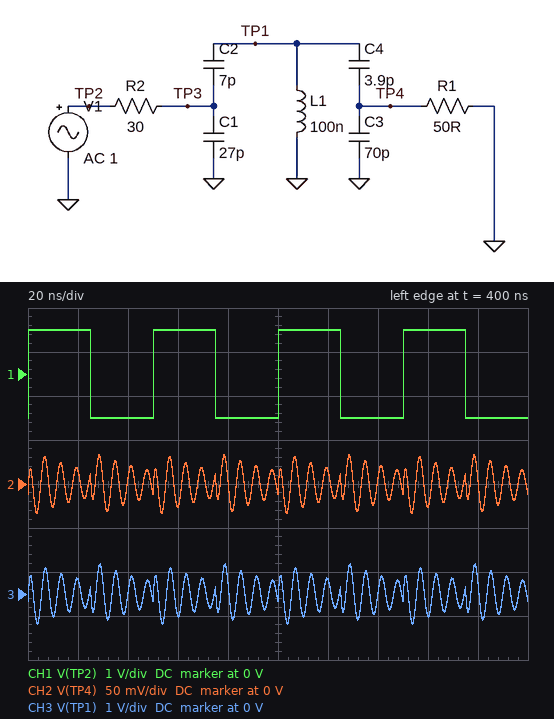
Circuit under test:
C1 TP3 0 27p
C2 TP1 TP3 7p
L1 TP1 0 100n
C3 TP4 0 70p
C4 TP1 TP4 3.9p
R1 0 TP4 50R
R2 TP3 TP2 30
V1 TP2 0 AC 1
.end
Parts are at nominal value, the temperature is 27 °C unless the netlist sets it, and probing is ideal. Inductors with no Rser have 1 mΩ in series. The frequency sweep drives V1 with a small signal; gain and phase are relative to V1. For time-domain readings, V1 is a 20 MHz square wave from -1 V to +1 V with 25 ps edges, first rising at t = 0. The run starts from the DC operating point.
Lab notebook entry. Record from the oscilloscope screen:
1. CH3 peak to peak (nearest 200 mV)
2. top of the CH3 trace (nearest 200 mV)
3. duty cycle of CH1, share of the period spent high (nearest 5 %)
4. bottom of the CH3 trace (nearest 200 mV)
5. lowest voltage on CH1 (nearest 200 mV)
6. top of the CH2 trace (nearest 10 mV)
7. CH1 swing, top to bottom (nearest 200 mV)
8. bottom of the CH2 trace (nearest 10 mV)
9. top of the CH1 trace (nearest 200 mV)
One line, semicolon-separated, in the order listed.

1.4 V; 600 mV; 50 %; -600 mV; -1.0 V; 30 mV; 2.0 V; -30 mV; 1.0 V
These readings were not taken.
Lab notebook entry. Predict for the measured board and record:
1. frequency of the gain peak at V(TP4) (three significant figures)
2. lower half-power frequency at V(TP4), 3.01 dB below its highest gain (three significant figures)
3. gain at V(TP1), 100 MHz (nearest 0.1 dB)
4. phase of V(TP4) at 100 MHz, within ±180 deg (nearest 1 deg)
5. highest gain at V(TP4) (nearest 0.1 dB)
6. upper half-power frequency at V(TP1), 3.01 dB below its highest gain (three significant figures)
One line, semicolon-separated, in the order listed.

159 MHz; 153 MHz; -8.1 dB; 168 deg; -9.8 dB; 166 MHz
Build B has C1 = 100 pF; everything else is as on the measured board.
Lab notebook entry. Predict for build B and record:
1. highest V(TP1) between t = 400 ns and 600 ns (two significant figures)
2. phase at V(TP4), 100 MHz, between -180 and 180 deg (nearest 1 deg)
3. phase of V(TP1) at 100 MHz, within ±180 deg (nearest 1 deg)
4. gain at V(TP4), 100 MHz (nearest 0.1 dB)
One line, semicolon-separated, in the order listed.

270 mV; 139 deg; 115 deg; -39.9 dB
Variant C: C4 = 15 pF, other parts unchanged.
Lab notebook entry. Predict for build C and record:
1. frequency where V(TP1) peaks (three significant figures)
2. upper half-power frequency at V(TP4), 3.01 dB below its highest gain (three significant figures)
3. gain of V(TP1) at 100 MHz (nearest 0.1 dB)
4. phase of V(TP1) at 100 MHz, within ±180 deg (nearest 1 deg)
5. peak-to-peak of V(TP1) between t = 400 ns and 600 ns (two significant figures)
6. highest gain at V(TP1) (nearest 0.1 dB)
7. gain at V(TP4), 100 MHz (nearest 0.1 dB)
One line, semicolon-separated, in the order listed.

115 MHz; 120 MHz; -0.5 dB; 133 deg; 790 mV; 11.7 dB; -16.2 dB
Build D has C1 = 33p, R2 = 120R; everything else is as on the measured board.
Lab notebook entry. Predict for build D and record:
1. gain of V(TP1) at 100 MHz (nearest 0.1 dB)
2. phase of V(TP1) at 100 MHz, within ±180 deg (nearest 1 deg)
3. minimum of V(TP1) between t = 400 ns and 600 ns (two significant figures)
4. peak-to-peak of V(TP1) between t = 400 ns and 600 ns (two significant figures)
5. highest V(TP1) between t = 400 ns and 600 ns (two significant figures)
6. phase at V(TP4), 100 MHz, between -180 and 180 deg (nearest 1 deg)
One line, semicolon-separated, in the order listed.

-17.1 dB; 107 deg; -190 mV; 380 mV; 190 mV; 130 deg
